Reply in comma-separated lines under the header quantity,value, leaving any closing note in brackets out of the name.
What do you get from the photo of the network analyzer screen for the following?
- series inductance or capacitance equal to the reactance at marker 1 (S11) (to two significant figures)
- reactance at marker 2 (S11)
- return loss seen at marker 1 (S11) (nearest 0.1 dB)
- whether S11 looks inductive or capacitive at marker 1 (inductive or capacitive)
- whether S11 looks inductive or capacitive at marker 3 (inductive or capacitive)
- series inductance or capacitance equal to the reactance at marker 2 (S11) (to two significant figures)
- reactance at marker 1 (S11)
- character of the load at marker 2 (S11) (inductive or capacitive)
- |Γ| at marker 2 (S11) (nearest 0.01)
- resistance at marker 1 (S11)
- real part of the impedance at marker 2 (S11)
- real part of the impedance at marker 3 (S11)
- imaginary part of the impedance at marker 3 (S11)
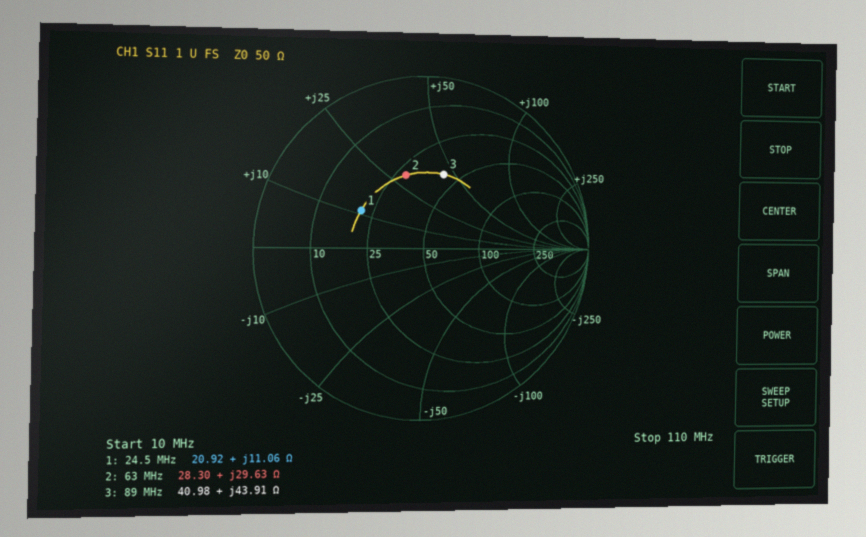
quantity,value
series inductance or capacitance equal to the reactance at marker 1 (S11),72 nH
reactance at marker 2,+29.63 Ω
return loss seen at marker 1 (S11),7.3 dB
whether S11 looks inductive or capacitive at marker 1,inductive
whether S11 looks inductive or capacitive at marker 3,inductive
series inductance or capacitance equal to the reactance at marker 2 (S11),75 nH
reactance at marker 1,+11.06 Ω
character of the load at marker 2 (S11),inductive
|Γ| at marker 2 (S11),0.44
resistance at marker 1,20.92 Ω
real part of the impedance at marker 2,28.30 Ω
real part of the impedance at marker 3,40.98 Ω
imaginary part of the impedance at marker 3,+43.91 Ω
